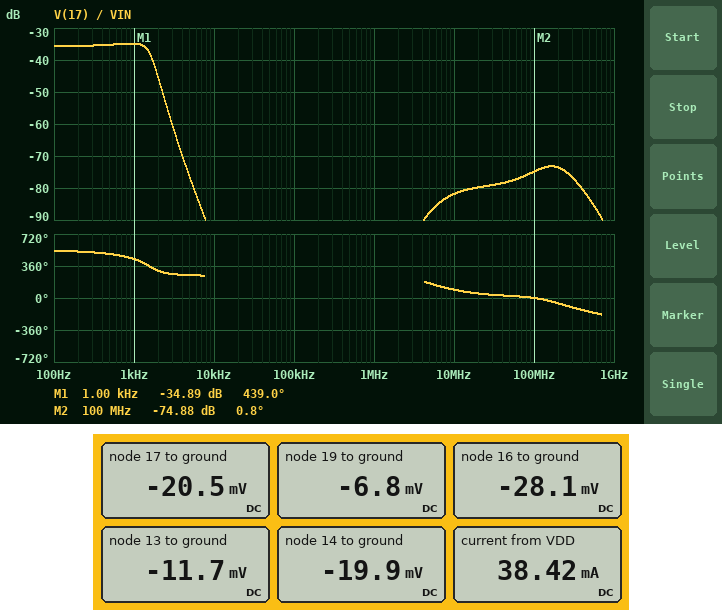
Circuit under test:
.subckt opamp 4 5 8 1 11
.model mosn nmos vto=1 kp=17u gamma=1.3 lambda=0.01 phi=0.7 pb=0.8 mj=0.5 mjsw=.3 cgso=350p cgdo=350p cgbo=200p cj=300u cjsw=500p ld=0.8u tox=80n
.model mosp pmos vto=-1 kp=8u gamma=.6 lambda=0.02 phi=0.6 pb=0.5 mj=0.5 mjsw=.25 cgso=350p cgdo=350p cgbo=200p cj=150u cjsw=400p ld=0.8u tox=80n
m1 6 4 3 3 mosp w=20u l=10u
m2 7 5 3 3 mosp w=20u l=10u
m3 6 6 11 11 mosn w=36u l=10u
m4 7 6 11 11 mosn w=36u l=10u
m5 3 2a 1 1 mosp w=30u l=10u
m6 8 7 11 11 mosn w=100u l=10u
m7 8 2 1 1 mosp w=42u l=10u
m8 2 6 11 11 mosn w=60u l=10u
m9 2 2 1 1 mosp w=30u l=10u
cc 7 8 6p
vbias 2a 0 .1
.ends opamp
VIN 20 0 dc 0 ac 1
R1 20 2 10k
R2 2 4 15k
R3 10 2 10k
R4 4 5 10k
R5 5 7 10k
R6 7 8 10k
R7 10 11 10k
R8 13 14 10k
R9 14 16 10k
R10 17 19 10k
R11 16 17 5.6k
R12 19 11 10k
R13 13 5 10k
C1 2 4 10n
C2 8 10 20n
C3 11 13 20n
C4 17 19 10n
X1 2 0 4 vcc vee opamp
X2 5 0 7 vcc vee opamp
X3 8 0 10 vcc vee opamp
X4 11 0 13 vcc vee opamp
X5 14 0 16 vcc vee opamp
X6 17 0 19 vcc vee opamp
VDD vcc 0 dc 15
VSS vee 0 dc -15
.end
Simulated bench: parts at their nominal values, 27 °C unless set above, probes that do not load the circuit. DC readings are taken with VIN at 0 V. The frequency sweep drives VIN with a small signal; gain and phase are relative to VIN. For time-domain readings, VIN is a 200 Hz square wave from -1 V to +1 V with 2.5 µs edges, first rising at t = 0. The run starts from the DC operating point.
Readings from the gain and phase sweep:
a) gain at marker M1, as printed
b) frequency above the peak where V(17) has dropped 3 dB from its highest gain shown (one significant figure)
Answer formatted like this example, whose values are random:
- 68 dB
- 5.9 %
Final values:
- -34.89 dB
- 2 kHz
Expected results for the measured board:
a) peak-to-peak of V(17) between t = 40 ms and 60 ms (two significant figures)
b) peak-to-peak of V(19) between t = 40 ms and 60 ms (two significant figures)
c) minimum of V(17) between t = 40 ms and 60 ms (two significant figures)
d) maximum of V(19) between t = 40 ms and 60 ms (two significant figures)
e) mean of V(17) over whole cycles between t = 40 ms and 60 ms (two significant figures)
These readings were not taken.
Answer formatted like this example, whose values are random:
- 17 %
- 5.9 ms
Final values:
- 45 mV
- 1.8 V
- -43 mV
- 880 mV
- -21 mV
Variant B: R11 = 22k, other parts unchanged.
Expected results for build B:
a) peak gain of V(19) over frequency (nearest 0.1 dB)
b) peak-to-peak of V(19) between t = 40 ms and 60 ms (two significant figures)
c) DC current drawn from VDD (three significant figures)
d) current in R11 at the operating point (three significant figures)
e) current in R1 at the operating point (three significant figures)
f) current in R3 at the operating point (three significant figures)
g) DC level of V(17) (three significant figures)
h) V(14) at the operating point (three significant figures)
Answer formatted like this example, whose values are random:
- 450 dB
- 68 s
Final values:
- -9.1 dB
- 790 mV
- 38.4 mA
- 724 nA
- 1.98 µA
- 824 nA
- -20.3 mV
- -19.8 mV
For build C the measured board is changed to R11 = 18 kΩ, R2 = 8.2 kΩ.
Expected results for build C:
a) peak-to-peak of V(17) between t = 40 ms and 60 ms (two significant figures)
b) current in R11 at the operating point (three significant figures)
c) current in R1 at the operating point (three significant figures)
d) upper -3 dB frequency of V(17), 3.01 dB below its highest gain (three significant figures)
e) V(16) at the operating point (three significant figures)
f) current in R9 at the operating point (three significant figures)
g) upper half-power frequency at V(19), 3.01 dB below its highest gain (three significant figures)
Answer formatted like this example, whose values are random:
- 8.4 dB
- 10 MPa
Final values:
- 18 mV
- 562 nA
- 1.98 µA
- 1.20 kHz
- -30.4 mV
- 1.05 µA
- 1.19 kHz
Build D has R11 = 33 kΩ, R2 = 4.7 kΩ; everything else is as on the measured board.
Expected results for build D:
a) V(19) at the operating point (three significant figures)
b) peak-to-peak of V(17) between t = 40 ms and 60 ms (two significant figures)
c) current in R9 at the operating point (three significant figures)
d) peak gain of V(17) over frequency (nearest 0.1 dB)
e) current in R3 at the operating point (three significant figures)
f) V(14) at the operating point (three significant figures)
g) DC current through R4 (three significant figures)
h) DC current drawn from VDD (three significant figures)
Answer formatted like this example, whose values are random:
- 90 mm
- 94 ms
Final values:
- -18.0 mV
- 8.7 mV
- 753 nA
- -47.8 dB
- 282 nA
- -20.0 mV
- 773 nA
- 38.4 mA
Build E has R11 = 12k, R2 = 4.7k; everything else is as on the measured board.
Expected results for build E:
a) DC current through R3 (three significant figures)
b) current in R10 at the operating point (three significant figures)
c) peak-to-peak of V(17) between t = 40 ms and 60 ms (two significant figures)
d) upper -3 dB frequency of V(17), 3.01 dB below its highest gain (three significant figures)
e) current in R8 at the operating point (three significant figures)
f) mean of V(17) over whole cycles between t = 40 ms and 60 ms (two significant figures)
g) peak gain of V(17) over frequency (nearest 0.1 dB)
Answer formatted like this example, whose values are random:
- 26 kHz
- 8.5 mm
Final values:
- 544 nA
- 502 nA
- 16 mV
- 1.19 kHz
- 629 nA
- -20 mV
- -43.5 dB
